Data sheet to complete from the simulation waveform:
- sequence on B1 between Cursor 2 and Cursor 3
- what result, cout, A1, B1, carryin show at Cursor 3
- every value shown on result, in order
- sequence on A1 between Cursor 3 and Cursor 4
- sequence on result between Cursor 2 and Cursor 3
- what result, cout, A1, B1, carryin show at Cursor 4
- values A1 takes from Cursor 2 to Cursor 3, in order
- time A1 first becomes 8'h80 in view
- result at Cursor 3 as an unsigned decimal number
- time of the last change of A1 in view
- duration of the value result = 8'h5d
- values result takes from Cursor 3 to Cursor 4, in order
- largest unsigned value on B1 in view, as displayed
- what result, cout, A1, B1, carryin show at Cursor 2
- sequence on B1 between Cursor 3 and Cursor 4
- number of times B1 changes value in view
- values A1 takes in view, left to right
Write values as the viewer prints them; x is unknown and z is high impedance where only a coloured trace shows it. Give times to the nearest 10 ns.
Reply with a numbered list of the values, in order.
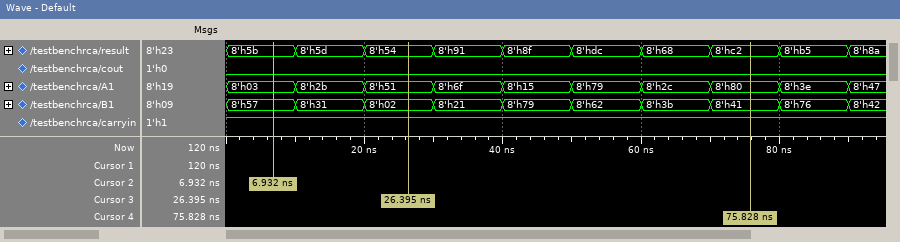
1. 8'h57, 8'h31, 8'h02
2. result=8'h54, cout=0, A1=8'h51, B1=8'h02, carryin=1
3. 8'h5b, 8'h5d, 8'h54, 8'h91, 8'h8f, 8'hdc, 8'h68, 8'hc2, 8'hb5, 8'h8a
4. 8'h51, 8'h6f, 8'h15, 8'h79, 8'h2c, 8'h80
5. 8'h5b, 8'h5d, 8'h54
6. result=8'hc2, cout=0, A1=8'h80, B1=8'h41, carryin=1
7. 8'h03, 8'h2b, 8'h51
8. 70 ns
9. 84
10. 90 ns
11. 10 ns
12. 8'h54, 8'h91, 8'h8f, 8'hdc, 8'h68, 8'hc2
13. 8'h79
14. result=8'h5b, cout=0, A1=8'h03, B1=8'h57, carryin=1
15. 8'h02, 8'h21, 8'h79, 8'h62, 8'h3b, 8'h41
16. 9
17. 8'h03, 8'h2b, 8'h51, 8'h6f, 8'h15, 8'h79, 8'h2c, 8'h80, 8'h3e, 8'h47
